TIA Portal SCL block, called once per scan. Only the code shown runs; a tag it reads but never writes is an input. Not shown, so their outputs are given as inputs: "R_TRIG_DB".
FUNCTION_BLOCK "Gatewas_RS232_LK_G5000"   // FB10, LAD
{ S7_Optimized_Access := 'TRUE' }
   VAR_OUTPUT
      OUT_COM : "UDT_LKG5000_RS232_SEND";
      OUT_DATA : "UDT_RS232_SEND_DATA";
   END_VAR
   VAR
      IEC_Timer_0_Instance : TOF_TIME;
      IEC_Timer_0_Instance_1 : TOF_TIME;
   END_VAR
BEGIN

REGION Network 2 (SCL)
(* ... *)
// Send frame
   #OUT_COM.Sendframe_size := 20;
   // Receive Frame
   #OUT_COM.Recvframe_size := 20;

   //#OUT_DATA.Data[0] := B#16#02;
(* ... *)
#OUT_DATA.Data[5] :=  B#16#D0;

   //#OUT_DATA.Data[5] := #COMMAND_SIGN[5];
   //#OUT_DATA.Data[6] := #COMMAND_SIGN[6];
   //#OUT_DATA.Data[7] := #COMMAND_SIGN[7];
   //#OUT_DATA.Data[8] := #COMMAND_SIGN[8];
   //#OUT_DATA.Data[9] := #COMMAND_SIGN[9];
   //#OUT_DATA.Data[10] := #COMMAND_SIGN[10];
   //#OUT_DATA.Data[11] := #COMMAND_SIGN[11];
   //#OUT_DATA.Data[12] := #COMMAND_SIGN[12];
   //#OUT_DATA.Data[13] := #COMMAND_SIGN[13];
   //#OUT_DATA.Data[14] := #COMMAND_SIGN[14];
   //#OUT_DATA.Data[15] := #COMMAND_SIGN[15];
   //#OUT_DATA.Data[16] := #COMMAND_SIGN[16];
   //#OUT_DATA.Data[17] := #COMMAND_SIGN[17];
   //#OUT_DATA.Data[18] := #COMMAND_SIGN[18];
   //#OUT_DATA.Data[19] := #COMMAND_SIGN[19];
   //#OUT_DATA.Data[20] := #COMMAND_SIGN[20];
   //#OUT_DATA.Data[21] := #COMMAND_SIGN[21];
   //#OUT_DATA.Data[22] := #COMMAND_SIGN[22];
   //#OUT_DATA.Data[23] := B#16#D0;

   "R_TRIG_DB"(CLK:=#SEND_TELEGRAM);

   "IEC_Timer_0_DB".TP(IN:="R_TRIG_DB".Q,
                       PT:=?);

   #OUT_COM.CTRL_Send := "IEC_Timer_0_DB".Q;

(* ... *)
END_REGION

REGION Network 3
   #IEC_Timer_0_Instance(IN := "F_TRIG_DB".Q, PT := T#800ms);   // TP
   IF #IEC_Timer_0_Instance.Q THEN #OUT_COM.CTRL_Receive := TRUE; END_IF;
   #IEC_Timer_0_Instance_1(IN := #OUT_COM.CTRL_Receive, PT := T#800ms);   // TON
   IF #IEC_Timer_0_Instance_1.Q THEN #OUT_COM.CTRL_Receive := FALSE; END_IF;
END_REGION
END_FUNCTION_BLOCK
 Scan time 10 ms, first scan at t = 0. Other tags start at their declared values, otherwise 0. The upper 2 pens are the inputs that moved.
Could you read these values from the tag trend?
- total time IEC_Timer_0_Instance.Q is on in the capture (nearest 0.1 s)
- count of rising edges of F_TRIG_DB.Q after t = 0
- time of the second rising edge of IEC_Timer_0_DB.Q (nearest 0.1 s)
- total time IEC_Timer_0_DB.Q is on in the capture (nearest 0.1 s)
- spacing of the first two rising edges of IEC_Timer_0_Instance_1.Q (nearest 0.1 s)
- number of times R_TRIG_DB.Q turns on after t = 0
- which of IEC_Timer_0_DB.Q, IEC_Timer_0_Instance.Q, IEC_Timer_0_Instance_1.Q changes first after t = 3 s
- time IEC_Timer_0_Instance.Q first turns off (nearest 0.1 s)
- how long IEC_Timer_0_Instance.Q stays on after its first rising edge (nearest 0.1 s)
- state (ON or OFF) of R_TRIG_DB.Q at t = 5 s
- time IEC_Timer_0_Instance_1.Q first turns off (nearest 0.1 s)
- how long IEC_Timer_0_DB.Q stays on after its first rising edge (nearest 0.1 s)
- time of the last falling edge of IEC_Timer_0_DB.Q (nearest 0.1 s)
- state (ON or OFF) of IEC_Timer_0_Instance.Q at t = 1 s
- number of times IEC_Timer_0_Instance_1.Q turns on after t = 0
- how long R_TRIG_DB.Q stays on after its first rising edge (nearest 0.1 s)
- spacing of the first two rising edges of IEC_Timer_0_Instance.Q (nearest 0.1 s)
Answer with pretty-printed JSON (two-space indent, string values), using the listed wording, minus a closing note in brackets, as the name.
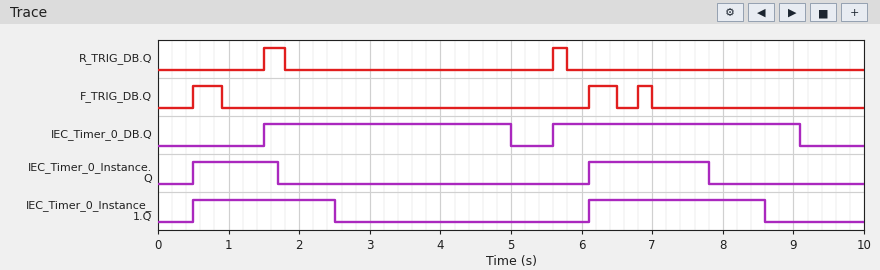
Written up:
{
  "total time IEC_Timer_0_Instance.Q is on in the capture": "2.9 s",
  "count of rising edges of F_TRIG_DB.Q after t = 0": "3",
  "time of the second rising edge of IEC_Timer_0_DB.Q": "5.6 s",
  "total time IEC_Timer_0_DB.Q is on in the capture": "7.0 s",
  "spacing of the first two rising edges of IEC_Timer_0_Instance_1.Q": "5.6 s",
  "number of times R_TRIG_DB.Q turns on after t = 0": "2",
  "which of IEC_Timer_0_DB.Q, IEC_Timer_0_Instance.Q, IEC_Timer_0_Instance_1.Q changes first after t = 3 s": "IEC_Timer_0_DB.Q",
  "time IEC_Timer_0_Instance.Q first turns off": "1.7 s",
  "how long IEC_Timer_0_Instance.Q stays on after its first rising edge": "1.2 s",
  "state (ON or OFF) of R_TRIG_DB.Q at t = 5 s": "OFF",
  "time IEC_Timer_0_Instance_1.Q first turns off": "2.5 s",
  "how long IEC_Timer_0_DB.Q stays on after its first rising edge": "3.5 s",
  "time of the last falling edge of IEC_Timer_0_DB.Q": "9.1 s",
  "state (ON or OFF) of IEC_Timer_0_Instance.Q at t = 1 s": "ON",
  "number of times IEC_Timer_0_Instance_1.Q turns on after t = 0": "2",
  "how long R_TRIG_DB.Q stays on after its first rising edge": "0.3 s",
  "spacing of the first two rising edges of IEC_Timer_0_Instance.Q": "5.6 s"
}
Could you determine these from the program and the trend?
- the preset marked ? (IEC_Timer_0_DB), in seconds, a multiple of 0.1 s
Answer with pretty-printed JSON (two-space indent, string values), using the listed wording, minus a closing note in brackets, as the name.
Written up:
{
  "the preset marked ? (IEC_Timer_0_DB), in seconds, a multiple of 0.1 s": "3.5 s"
}
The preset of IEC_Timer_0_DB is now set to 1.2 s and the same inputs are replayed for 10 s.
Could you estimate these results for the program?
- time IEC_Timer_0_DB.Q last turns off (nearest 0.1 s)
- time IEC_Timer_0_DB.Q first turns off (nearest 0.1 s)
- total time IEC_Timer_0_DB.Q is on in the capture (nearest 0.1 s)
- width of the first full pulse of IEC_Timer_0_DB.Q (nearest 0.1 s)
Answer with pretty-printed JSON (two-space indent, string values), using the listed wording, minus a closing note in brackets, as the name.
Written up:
{
  "time IEC_Timer_0_DB.Q last turns off": "6.8 s",
  "time IEC_Timer_0_DB.Q first turns off": "2.7 s",
  "total time IEC_Timer_0_DB.Q is on in the capture": "2.4 s",
  "width of the first full pulse of IEC_Timer_0_DB.Q": "1.2 s"
}
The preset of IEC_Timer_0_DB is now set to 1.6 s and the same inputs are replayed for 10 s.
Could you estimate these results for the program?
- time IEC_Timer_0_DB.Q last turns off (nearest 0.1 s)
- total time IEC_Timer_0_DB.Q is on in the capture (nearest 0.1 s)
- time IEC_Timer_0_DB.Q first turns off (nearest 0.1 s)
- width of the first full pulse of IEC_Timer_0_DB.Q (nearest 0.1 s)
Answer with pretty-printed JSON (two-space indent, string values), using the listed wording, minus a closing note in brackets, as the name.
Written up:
{
  "time IEC_Timer_0_DB.Q last turns off": "7.2 s",
  "total time IEC_Timer_0_DB.Q is on in the capture": "3.2 s",
  "time IEC_Timer_0_DB.Q first turns off": "3.1 s",
  "width of the first full pulse of IEC_Timer_0_DB.Q": "1.6 s"
}
